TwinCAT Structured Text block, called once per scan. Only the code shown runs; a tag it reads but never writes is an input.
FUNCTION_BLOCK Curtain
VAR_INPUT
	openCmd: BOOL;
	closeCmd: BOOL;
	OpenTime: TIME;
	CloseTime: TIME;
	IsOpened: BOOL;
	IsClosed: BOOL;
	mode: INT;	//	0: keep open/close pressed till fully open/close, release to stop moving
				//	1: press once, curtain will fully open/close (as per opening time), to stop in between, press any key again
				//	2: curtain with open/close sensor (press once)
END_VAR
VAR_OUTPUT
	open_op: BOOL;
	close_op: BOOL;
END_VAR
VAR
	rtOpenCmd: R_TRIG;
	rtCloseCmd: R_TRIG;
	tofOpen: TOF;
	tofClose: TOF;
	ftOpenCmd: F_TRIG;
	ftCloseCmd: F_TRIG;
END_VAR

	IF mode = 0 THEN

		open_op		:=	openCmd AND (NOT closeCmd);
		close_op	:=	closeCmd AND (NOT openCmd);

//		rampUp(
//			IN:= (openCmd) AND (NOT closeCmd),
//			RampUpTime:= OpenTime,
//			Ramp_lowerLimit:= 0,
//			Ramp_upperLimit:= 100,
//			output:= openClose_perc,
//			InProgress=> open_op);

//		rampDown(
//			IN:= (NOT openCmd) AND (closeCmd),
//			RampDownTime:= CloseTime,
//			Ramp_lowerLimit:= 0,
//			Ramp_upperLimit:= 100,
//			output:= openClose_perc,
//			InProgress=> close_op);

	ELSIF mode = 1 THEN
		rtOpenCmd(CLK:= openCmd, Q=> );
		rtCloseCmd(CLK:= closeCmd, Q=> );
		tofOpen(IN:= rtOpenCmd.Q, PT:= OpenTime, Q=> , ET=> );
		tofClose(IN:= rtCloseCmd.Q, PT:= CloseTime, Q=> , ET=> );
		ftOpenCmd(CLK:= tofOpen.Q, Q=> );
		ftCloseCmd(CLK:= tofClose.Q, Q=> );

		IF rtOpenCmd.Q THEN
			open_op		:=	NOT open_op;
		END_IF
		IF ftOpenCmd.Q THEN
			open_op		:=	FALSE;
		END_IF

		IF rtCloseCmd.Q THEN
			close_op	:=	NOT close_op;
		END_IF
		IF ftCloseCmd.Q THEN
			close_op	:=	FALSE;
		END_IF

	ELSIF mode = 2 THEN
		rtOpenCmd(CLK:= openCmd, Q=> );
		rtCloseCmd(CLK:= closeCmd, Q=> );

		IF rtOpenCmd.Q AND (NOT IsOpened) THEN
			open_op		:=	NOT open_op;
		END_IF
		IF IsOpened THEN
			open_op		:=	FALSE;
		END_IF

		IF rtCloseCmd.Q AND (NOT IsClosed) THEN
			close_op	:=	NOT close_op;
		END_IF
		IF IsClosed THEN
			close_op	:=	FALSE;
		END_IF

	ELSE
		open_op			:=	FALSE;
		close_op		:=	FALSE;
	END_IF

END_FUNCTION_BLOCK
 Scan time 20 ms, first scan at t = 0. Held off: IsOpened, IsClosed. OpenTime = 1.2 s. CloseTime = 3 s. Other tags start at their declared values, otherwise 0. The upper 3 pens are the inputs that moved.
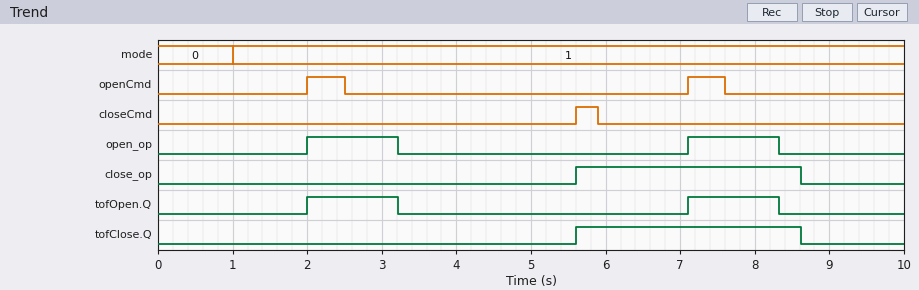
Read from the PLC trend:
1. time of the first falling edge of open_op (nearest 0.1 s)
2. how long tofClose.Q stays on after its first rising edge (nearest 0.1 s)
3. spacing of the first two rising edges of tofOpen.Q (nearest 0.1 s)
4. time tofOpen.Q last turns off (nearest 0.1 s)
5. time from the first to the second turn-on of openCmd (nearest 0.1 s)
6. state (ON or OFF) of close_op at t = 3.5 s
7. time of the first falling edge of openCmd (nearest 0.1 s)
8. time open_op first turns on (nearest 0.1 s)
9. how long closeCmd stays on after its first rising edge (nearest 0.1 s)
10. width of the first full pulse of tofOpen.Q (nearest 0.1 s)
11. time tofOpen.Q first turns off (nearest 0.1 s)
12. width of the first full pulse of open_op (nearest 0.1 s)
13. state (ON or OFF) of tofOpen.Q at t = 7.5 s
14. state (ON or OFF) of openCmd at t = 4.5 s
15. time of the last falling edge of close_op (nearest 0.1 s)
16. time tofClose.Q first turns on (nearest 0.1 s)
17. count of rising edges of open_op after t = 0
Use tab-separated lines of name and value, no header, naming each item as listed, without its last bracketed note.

time of the first falling edge of open_op	3.2 s
how long tofClose.Q stays on after its first rising edge	3.0 s
spacing of the first two rising edges of tofOpen.Q	5.1 s
time tofOpen.Q last turns off	8.3 s
time from the first to the second turn-on of openCmd	5.1 s
state (ON or OFF) of close_op at t = 3.5 s	OFF
time of the first falling edge of openCmd	2.5 s
time open_op first turns on	2.0 s
how long closeCmd stays on after its first rising edge	0.3 s
width of the first full pulse of tofOpen.Q	1.2 s
time tofOpen.Q first turns off	3.2 s
width of the first full pulse of open_op	1.2 s
state (ON or OFF) of tofOpen.Q at t = 7.5 s	ON
state (ON or OFF) of openCmd at t = 4.5 s	OFF
time of the last falling edge of close_op	8.6 s
time tofClose.Q first turns on	5.6 s
count of rising edges of open_op after t = 0	2
